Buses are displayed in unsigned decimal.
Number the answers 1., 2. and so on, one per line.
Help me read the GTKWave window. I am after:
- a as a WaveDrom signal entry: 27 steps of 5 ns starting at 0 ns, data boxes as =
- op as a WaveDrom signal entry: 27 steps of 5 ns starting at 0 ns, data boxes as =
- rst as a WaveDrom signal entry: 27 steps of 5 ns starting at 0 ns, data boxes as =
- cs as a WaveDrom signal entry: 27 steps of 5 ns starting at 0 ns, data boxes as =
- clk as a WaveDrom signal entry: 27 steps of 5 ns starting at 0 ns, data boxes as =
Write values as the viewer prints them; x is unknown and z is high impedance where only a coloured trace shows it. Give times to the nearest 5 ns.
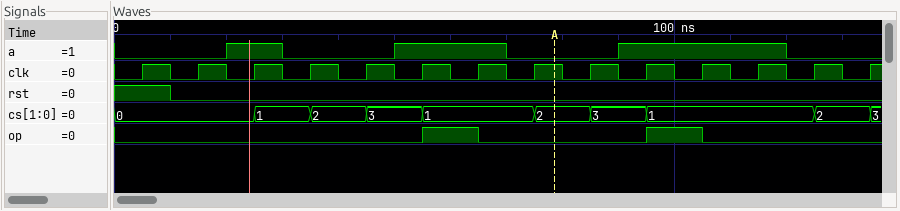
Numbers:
1. {name: 'a', wave: '0...1.0...1...0...1.....0..'}
2. {name: 'op', wave: '0..........1.0.....1.0.....'}
3. {name: 'rst', wave: '1.0........................'}
4. {name: 'cs', wave: '=....=.=.=.=...=.=.=.....=.', data: '0 1 2 3 1 2 3 1 2'}
5. {name: 'clk', wave: '010101010101010101010101010'}
